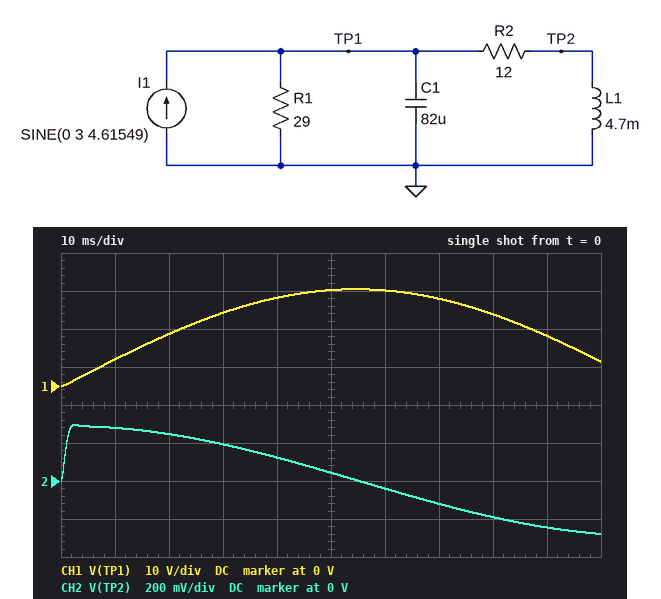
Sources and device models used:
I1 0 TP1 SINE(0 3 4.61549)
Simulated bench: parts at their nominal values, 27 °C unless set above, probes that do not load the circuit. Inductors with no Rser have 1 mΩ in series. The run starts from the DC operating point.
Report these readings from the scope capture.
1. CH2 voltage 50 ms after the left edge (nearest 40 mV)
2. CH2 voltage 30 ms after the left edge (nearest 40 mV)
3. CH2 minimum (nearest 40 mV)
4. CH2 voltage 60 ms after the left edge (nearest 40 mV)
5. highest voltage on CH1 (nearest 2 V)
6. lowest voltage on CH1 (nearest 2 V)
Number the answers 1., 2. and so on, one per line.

1. 40 mV
2. 200 mV
3. -280 mV
4. -40 mV
5. 26 V
6. 0 V
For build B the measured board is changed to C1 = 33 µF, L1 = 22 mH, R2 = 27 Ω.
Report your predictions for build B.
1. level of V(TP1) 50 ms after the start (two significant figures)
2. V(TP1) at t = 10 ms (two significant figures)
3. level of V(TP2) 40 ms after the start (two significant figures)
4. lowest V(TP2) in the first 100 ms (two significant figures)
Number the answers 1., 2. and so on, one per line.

1. 42 V
2. 12 V
3. 420 mV
4. -960 mV
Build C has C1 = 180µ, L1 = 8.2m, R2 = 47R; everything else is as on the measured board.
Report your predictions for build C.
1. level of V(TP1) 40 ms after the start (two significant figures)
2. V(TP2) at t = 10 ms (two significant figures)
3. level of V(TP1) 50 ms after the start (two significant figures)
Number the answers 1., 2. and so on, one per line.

1. 47 V
2. 250 mV
3. 52 V
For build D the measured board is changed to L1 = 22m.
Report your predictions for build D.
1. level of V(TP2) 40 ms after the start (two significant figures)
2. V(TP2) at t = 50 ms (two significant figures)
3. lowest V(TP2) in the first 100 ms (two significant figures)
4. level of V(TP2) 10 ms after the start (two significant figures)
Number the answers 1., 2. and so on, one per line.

1. 590 mV
2. 210 mV
3. -1.3 V
4. 1.3 V
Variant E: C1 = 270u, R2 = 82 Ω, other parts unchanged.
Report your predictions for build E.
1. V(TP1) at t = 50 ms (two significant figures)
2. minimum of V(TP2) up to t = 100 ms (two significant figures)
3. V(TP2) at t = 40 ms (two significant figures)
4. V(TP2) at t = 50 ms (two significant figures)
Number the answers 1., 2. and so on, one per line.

1. 61 V
2. -96 mV
3. 58 mV
4. 31 mV
